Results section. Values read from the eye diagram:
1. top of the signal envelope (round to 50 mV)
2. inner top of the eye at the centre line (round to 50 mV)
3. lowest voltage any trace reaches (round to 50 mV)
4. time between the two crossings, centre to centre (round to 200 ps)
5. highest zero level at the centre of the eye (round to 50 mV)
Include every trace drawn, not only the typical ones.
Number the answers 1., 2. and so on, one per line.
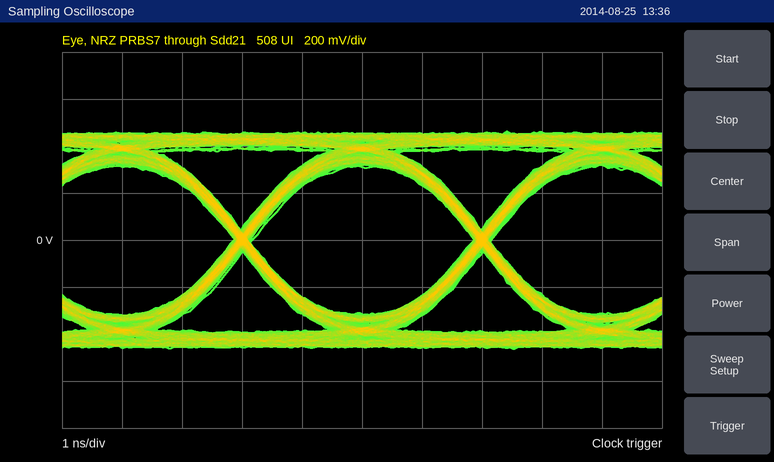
1. 450 mV
2. 300 mV
3. -450 mV
4. 4.0 ns
5. -300 mV
